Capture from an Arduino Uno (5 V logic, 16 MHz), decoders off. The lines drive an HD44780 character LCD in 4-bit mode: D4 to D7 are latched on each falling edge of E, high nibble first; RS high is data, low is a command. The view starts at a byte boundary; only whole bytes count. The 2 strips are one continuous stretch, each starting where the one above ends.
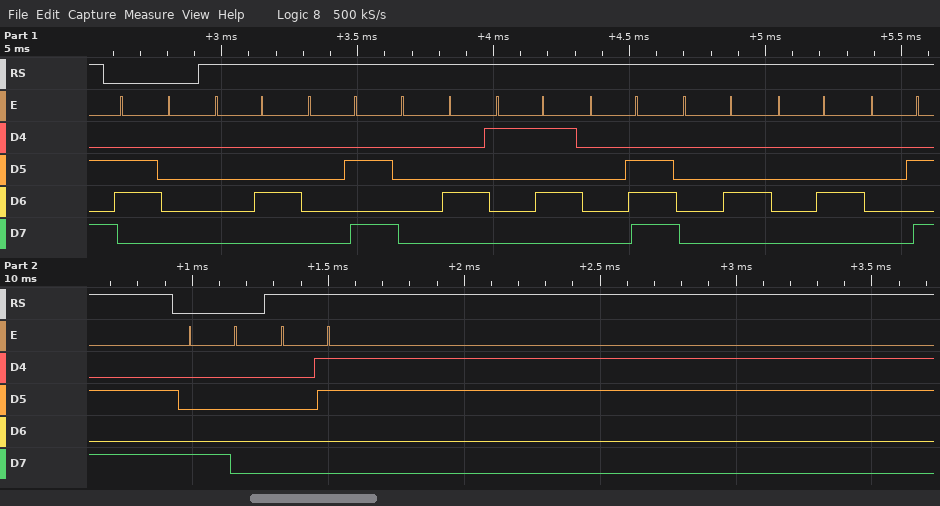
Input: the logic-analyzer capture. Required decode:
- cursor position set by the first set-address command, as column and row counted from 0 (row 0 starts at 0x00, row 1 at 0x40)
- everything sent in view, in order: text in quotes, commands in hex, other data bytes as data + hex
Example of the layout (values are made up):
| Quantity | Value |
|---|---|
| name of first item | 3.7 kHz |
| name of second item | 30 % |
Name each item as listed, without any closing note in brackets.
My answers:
| Quantity | Value |
|---|---|
| cursor position set by the first set-address command, as column and row counted from 0 | column 0, row 0 |
| everything sent in view, in order: text in quotes, commands in hex, other data bytes as data + hex | 0x60 data 04 0A 04 15 0E 04 04 0A 0x80 data 03 |
